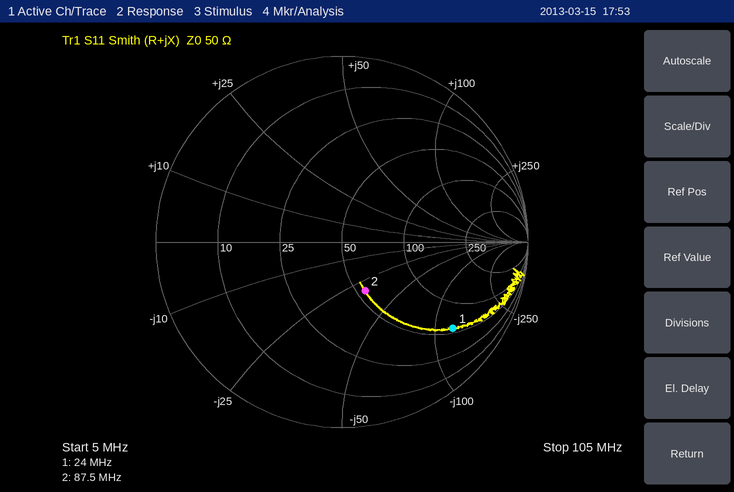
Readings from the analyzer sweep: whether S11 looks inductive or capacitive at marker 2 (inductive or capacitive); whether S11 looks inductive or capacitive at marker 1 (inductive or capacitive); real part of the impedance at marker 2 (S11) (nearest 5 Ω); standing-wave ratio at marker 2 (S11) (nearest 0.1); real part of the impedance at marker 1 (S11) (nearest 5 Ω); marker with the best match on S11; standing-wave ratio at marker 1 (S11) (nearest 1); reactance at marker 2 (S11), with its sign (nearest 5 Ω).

capacitive
capacitive
55 Ω
1.8
55 Ω
marker 2
7
-30 Ω
